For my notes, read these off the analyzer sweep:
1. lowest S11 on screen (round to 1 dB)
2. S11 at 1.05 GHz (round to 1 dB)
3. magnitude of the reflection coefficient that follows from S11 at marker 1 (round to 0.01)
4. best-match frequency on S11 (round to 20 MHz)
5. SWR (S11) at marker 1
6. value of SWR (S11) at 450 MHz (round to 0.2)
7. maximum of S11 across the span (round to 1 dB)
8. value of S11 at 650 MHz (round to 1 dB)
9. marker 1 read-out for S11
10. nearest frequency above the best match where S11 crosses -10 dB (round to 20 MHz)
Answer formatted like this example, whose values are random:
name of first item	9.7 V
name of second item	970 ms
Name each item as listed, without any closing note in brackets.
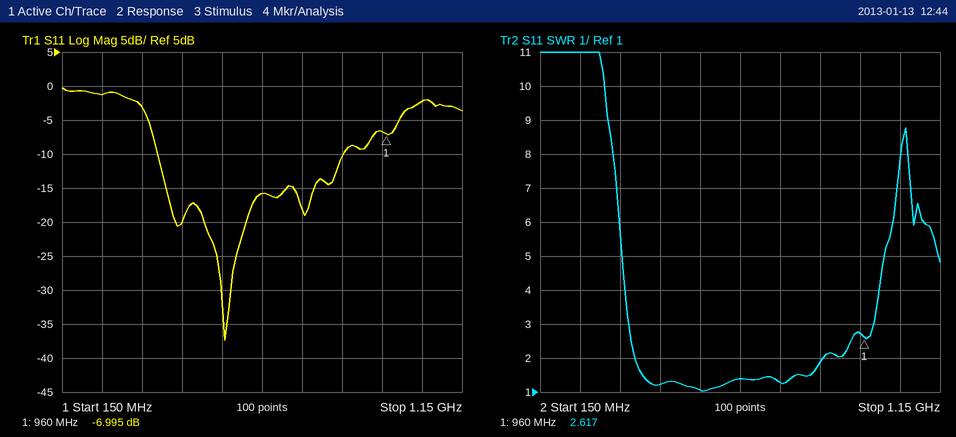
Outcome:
lowest S11 on screen	-37 dB
S11 at 1.05 GHz	-2 dB
magnitude of the reflection coefficient that follows from S11 at marker 1	0.45
best-match frequency on S11	560 MHz
SWR (S11) at marker 1	2.617
value of SWR (S11) at 450 MHz	1.2
maximum of S11 across the span	0 dB
value of S11 at 650 MHz	-16 dB
marker 1 read-out for S11	-6.995 dB
nearest frequency above the best match where S11 crosses -10 dB	860 MHz
